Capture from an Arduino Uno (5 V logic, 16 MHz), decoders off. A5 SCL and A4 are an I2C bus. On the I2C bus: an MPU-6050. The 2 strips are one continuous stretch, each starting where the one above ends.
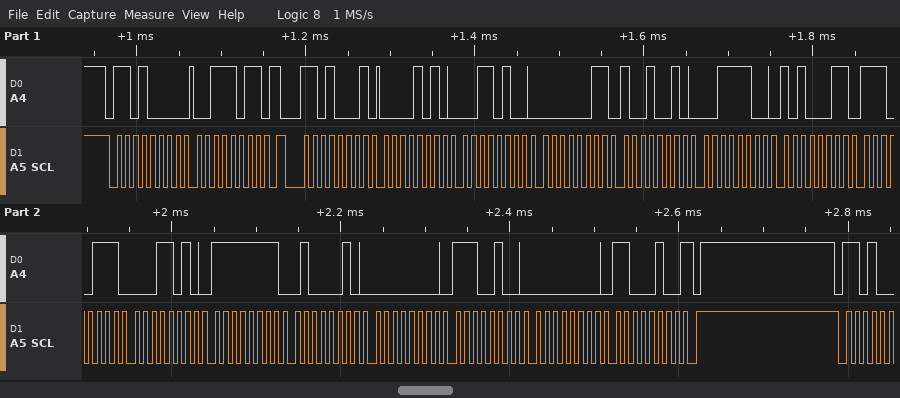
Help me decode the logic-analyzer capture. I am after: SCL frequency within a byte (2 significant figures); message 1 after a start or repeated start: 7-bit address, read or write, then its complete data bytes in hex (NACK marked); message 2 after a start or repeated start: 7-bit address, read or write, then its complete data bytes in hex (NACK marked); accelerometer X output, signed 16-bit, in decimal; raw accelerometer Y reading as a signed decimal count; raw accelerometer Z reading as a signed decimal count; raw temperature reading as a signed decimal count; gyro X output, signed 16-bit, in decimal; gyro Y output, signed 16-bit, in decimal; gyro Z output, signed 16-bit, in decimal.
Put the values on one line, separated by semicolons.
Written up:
100 kHz; 0x68 write: 3B; 0x68 read: 0A 34 03 92 3C A3 E7 1A FF 42 00 E4 00 C4 NACK; 2612; 914; 15523; -6374; -190; 228; 196
